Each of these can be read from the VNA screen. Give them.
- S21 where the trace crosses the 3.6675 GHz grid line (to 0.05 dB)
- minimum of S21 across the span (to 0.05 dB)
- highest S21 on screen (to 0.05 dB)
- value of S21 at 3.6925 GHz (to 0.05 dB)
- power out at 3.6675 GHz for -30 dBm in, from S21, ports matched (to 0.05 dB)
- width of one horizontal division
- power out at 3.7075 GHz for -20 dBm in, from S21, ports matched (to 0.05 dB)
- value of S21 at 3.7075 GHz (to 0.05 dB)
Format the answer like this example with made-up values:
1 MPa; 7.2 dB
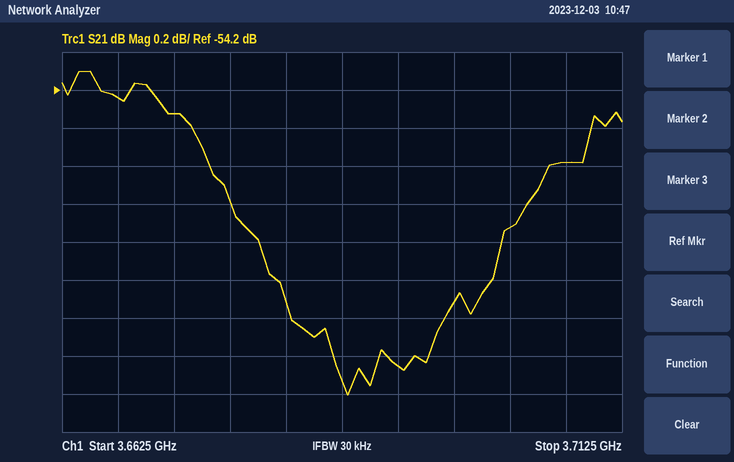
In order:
-54.25 dB; -55.80 dB; -54.10 dB; -55.65 dB; -84.25 dBm; 5 MHz; -74.60 dBm; -54.60 dB
